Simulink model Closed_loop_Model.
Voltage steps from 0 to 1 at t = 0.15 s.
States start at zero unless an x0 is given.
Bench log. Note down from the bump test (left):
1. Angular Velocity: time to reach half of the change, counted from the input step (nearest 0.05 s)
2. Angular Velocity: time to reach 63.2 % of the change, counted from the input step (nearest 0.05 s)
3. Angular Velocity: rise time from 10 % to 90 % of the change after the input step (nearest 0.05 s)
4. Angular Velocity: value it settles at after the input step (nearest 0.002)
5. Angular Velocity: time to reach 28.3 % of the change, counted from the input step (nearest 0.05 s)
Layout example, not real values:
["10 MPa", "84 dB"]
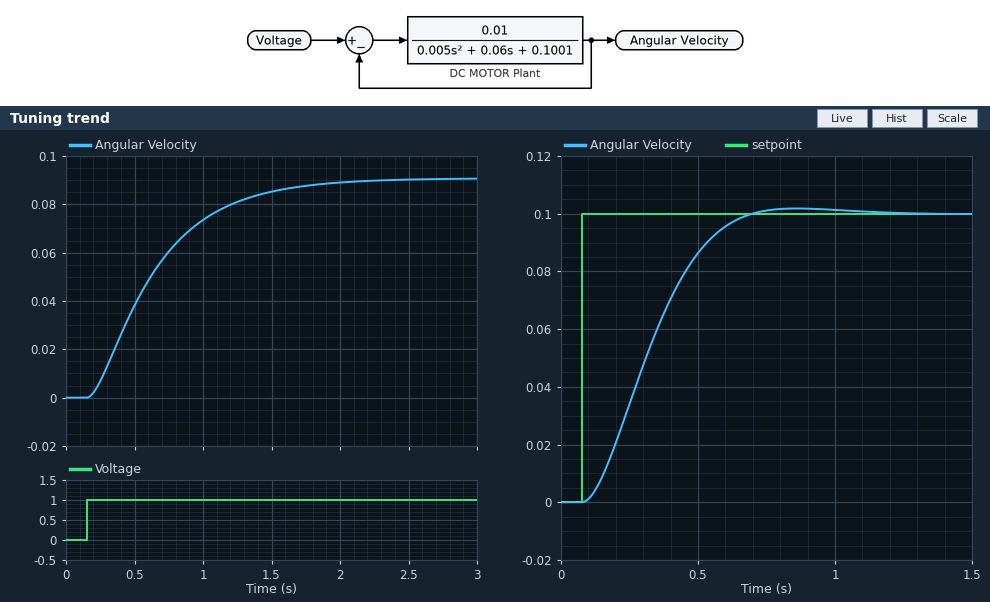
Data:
["0.40 s", "0.55 s", "1.00 s", "0.090", "0.25 s"]
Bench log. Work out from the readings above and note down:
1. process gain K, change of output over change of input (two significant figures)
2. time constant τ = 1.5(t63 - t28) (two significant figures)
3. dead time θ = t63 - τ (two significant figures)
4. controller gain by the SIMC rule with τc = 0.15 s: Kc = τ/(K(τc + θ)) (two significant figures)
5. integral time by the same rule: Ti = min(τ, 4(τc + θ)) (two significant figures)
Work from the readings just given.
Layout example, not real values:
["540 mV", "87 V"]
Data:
["0.090", "0.45 s", "0.10 s", "20", "0.45 s"]
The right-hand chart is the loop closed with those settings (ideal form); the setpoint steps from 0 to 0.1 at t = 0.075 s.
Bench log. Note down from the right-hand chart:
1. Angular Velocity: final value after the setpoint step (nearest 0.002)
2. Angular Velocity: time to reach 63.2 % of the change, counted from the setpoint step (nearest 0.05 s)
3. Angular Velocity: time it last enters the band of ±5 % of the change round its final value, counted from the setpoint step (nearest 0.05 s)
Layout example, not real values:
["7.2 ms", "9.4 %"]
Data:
["0.100", "0.30 s", "0.50 s"]
